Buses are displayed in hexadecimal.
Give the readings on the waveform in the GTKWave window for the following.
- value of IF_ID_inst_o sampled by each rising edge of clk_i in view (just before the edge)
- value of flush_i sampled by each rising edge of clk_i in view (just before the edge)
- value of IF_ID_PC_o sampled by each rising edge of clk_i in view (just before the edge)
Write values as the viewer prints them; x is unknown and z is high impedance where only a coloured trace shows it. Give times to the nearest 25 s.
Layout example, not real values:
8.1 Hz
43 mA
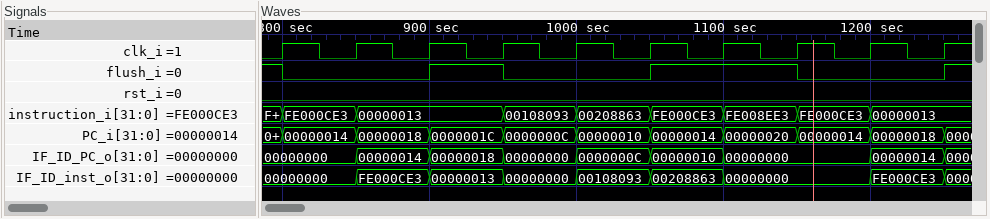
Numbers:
00000000, 00000000, FE000CE3, 00000013, 00000000, 00108093, 00208863, 00000000, 00000000, FE000CE3
1 0 0 1 0 0 1 1 0 0
00000000, 00000000, 00000014, 00000018, 00000000, 0000000C, 00000010, 00000000, 00000000, 00000014
